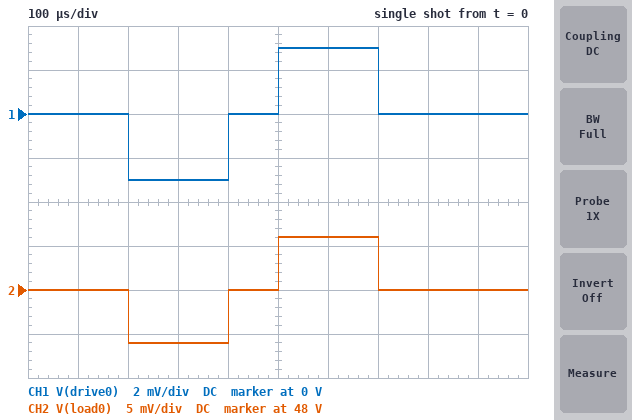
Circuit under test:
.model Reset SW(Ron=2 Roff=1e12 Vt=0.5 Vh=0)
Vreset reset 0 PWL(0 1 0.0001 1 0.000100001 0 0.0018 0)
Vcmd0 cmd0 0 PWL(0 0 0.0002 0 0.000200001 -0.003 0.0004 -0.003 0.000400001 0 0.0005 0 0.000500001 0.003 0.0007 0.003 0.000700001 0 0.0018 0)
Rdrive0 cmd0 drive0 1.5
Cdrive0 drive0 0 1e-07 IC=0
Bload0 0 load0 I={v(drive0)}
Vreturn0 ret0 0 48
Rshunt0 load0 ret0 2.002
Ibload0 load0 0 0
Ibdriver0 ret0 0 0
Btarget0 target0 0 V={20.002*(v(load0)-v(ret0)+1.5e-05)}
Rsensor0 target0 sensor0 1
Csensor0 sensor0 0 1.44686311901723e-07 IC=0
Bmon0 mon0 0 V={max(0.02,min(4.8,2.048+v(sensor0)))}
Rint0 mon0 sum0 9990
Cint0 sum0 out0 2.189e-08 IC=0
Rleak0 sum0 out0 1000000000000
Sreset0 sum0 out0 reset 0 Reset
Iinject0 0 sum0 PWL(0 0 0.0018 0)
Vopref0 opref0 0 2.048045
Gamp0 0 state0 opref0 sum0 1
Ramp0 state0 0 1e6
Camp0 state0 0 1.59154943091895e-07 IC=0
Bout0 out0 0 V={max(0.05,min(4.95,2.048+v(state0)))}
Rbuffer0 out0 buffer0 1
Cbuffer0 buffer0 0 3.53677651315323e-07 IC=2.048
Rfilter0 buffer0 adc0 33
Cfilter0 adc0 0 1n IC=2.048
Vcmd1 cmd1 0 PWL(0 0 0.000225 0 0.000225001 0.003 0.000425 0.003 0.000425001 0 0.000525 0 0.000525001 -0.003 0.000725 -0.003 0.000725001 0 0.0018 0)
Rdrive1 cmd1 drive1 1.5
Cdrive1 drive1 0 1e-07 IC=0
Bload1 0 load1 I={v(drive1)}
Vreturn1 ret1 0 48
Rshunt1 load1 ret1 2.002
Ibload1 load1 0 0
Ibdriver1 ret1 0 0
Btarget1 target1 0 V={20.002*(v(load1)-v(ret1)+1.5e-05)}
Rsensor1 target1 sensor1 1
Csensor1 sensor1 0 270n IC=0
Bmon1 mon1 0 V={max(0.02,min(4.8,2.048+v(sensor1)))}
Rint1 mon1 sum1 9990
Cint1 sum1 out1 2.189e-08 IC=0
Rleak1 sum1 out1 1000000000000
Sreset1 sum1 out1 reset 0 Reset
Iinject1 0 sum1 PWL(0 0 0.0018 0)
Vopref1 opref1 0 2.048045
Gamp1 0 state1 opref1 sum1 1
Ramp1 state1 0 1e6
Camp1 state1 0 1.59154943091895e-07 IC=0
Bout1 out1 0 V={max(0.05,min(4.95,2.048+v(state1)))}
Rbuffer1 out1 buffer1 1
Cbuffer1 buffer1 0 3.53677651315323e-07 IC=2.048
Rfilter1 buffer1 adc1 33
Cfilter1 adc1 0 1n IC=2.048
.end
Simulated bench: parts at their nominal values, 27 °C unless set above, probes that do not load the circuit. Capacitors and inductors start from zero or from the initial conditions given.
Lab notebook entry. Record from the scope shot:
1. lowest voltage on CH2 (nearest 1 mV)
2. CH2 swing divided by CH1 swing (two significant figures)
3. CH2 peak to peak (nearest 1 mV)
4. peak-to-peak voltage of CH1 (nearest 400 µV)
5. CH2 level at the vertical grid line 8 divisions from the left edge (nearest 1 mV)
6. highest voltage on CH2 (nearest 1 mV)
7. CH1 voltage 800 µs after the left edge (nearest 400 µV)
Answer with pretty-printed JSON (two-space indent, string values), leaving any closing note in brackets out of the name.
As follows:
{
  "lowest voltage on CH2": "47.994 V",
  "CH2 swing divided by CH1 swing": "2.0",
  "CH2 peak to peak": "12 mV",
  "peak-to-peak voltage of CH1": "6.0 mV",
  "CH2 level at the vertical grid line 8 divisions from the left edge": "48.000 V",
  "highest voltage on CH2": "48.006 V",
  "CH1 voltage 800 µs after the left edge": "0 V"
}
